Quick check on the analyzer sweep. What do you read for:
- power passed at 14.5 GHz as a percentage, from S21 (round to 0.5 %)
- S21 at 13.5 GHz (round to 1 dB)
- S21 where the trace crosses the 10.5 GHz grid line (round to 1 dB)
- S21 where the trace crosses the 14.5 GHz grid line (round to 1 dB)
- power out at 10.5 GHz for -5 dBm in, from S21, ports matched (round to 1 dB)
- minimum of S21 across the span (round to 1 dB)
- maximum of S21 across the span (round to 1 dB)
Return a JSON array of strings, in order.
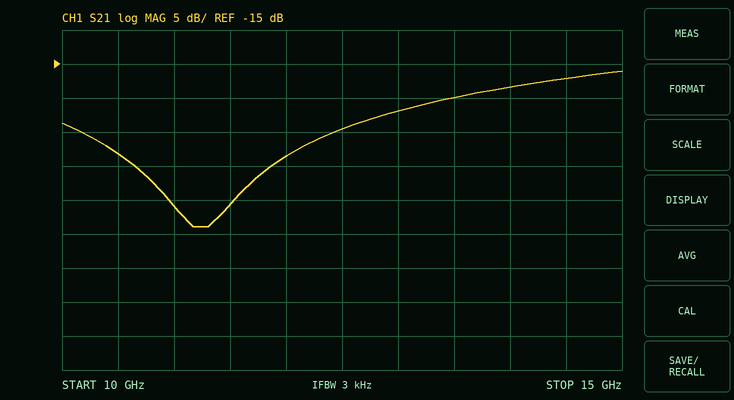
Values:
["2.0 %", "-20 dB", "-28 dB", "-17 dB", "-33 dBm", "-39 dB", "-16 dB"]
